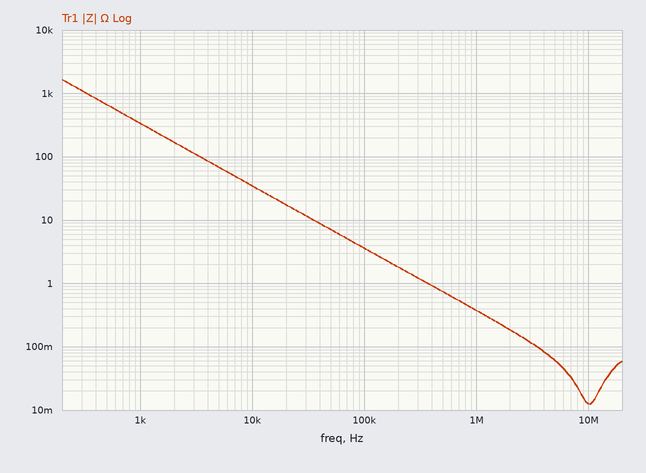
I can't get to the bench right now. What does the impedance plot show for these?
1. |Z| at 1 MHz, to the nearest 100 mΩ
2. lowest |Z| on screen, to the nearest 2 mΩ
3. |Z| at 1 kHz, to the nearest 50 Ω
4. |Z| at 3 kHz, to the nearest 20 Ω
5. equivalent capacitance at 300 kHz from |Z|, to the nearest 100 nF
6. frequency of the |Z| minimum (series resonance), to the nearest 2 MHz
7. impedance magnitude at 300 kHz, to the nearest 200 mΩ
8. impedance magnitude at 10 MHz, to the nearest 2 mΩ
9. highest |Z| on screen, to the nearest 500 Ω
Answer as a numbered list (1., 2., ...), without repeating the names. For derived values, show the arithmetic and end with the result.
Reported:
1. 400 mΩ
2. 12 mΩ
3. 350 Ω
4. 120 Ω
5. C = 1/(2π × 300 kHz × 1.2 Ω) ≈ 442 nF, so 400 nF to the nearest 100 nF
6. 10 MHz
7. 1.2 Ω
8. 12 mΩ
9. 1.5 kΩ
